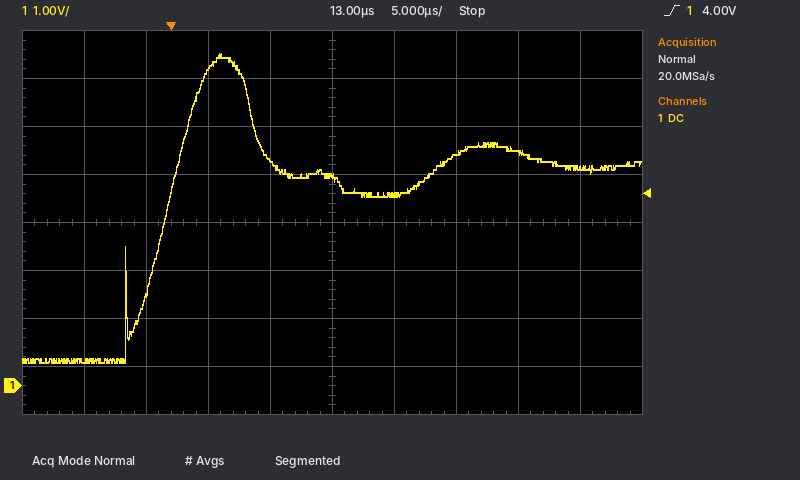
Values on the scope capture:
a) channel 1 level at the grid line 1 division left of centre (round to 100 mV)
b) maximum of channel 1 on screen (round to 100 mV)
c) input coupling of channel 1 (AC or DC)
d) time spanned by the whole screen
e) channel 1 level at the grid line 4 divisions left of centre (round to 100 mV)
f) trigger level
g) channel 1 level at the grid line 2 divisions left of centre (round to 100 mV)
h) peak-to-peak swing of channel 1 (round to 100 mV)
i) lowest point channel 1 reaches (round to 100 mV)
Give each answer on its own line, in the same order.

4.7 V
6.9 V
DC
50 µs
500 mV
4.00 V
6.6 V
6.4 V
500 mV
